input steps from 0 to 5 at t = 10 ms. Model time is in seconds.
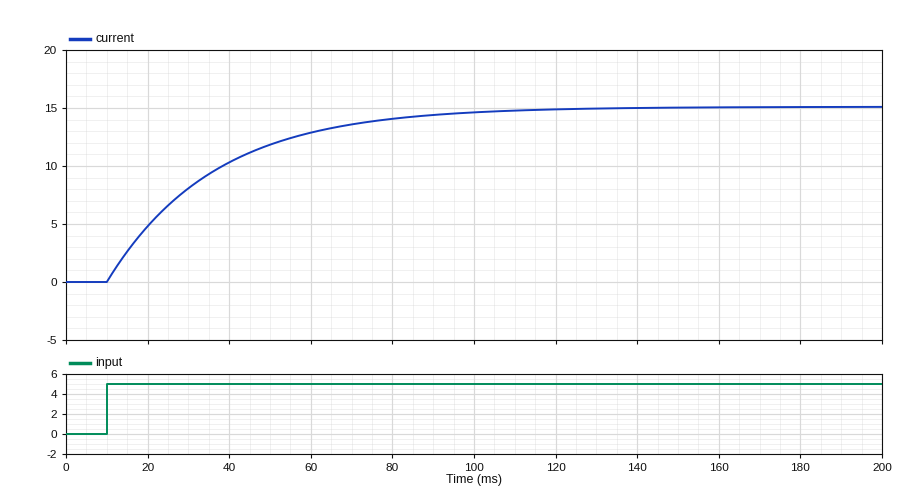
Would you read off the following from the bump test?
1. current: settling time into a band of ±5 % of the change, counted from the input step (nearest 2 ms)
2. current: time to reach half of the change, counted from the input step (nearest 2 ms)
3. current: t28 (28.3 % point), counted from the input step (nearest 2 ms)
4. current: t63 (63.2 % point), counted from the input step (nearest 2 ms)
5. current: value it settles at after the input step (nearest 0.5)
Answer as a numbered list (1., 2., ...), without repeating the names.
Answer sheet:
1. 78 ms
2. 18 ms
3. 8 ms
4. 26 ms
5. 15.0
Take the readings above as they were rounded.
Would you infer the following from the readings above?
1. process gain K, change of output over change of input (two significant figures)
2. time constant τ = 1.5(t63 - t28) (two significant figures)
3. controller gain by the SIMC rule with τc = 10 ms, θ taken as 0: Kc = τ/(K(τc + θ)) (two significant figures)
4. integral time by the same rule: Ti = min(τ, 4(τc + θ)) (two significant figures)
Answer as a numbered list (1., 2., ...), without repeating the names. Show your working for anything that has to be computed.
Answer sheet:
1. (15 - 0) / 5 = 3.0
2. 1.5 × (26 - 8) = 27 ms
3. 27 / (3 × (10 + 0)) = 0.90
4. min(27, 4 × (10 + 0)) = 27 ms
